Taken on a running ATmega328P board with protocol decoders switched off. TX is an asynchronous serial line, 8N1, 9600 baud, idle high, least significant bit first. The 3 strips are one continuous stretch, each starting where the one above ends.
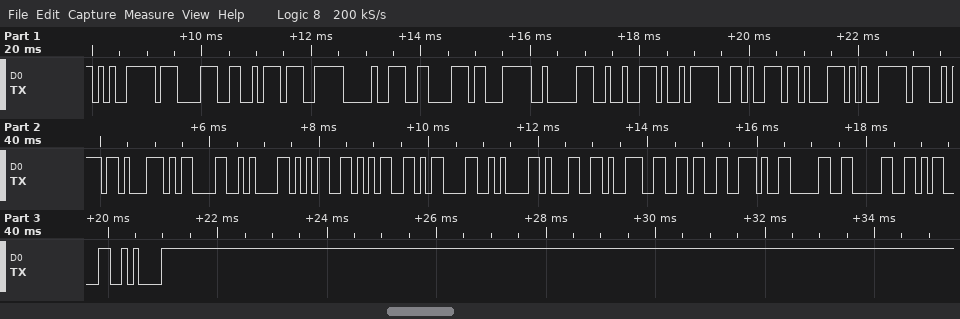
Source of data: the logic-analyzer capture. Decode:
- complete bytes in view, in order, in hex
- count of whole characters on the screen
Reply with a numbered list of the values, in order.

1. E5 87 A6 E7 90 86 E3 82 92 E9 96 8B E5 A7 8B 0D 0A 35 35 0D 0A 31 39 36 2E 30 30 0D 0A
2. 29
